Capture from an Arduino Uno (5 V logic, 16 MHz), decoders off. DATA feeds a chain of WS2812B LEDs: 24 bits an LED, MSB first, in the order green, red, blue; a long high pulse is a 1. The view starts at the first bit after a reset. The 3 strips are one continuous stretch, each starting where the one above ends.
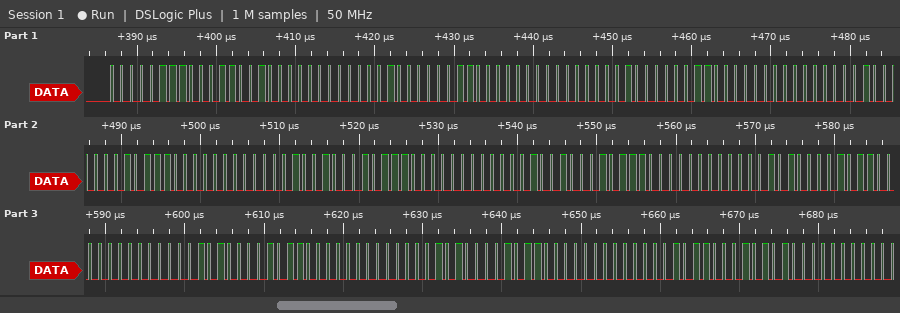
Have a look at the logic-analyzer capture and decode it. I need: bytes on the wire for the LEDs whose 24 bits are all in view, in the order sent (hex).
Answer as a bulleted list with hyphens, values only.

- 07 19 00 08 18 00 08 18 00 08 17 00 09 17 00 09 17 00 0A 16 00 0A 16 00 0A 16 00 0B 15 00
